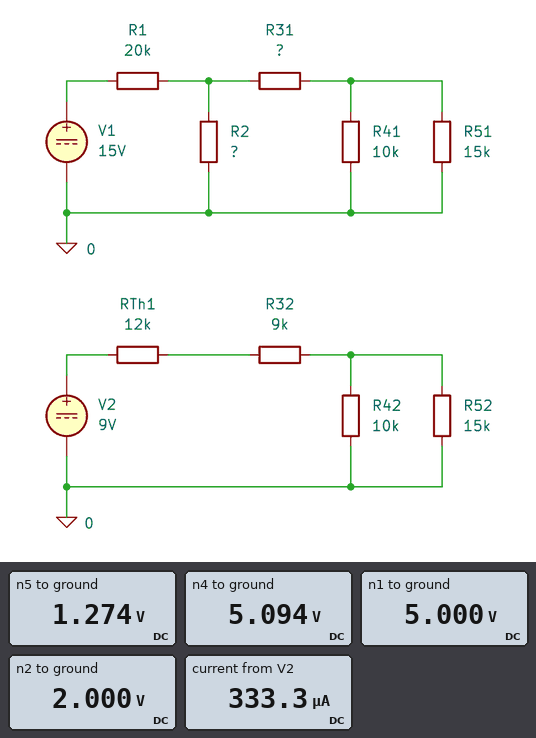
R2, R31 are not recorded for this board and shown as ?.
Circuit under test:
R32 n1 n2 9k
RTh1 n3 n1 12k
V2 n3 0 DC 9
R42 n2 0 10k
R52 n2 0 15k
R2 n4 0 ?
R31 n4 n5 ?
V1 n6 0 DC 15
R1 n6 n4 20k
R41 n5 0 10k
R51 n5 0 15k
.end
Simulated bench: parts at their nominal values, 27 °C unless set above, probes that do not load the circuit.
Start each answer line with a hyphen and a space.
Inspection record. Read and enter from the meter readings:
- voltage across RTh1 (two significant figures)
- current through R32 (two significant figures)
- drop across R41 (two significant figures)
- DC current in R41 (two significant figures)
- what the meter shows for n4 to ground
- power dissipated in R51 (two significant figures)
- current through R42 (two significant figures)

- 4.0 V
- 330 µA
- 1.3 V
- 130 µA
- 5.094 V
- 110 µW
- 200 µA
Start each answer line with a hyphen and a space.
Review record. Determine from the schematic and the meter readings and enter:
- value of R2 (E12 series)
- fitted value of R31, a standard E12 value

- 18 kΩ
- 18 kΩ
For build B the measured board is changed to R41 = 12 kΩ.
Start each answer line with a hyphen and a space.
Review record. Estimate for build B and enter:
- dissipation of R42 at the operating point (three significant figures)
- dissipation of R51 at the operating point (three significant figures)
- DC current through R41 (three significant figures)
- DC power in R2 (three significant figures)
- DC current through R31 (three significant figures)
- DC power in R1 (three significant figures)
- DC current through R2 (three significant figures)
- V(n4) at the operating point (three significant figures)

- 400 µW
- 128 µW
- 116 µA
- 1.46 mW
- 208 µA
- 4.87 mW
- 285 µA
- 5.13 V
